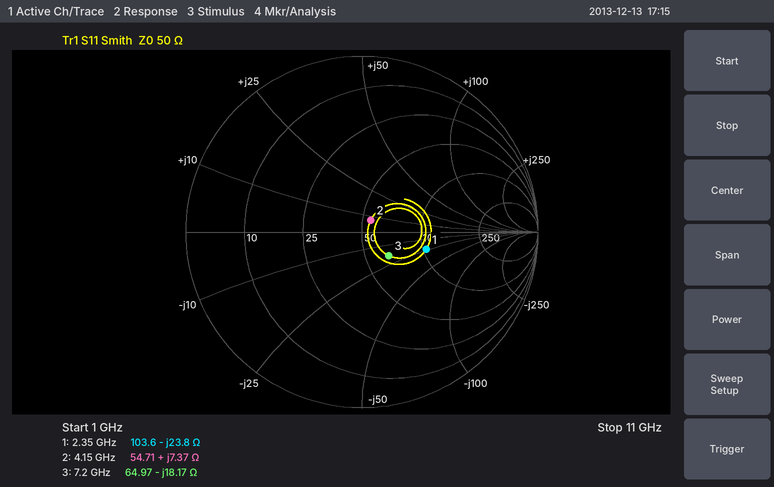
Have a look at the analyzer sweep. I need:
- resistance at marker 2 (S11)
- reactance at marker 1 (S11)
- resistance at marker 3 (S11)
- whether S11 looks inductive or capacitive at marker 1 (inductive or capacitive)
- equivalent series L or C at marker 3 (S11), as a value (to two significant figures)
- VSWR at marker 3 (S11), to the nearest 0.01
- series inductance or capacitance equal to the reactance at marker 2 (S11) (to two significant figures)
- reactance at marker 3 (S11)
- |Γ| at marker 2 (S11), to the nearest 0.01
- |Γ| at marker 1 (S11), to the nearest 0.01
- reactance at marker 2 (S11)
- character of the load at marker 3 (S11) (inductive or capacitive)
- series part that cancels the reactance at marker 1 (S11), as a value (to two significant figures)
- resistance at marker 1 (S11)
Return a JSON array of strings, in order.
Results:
["54.71 Ω", "-23.8 Ω", "64.97 Ω", "capacitive", "1.2 pF", "1.51", "280 pH", "-18.17 Ω", "0.08", "0.38", "+7.37 Ω", "capacitive", "1.6 nH", "103.6 Ω"]
